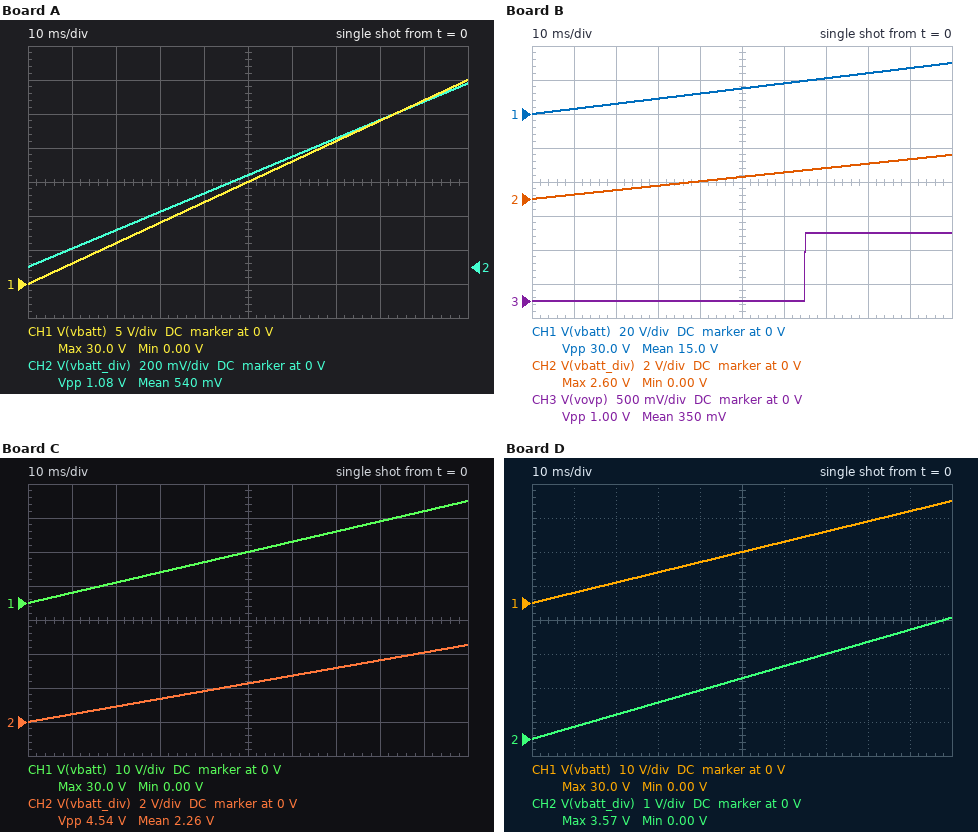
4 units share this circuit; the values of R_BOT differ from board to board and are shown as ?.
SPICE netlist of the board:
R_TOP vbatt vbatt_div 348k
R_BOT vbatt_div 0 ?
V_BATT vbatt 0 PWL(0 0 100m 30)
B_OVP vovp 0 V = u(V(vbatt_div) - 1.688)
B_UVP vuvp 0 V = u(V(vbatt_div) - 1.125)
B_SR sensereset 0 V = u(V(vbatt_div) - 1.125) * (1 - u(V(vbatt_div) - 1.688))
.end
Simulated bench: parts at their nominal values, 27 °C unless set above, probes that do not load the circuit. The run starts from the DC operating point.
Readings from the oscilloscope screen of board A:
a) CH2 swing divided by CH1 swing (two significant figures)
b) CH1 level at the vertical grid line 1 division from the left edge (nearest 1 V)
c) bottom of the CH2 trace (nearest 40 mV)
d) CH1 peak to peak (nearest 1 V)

0.036
3 V
0 V
30 V
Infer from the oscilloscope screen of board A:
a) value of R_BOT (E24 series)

13 kΩ
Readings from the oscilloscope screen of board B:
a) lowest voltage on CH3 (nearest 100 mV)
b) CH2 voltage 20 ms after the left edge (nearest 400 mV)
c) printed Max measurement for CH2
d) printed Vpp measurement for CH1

0 V
400 mV
2.60 V
30.0 V
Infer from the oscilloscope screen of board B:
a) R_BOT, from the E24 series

33 kΩ
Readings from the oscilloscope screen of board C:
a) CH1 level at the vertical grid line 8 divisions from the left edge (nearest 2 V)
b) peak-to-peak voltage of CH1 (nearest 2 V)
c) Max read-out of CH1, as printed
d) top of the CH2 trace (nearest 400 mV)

24 V
30 V
30.0 V
4.4 V
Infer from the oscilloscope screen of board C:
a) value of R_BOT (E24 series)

62 kΩ
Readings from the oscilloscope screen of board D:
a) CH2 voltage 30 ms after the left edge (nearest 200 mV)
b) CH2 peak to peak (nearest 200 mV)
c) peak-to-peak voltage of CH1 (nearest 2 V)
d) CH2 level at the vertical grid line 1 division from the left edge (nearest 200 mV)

1.0 V
3.6 V
30 V
400 mV
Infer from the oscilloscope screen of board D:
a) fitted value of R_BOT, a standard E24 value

47 kΩ
